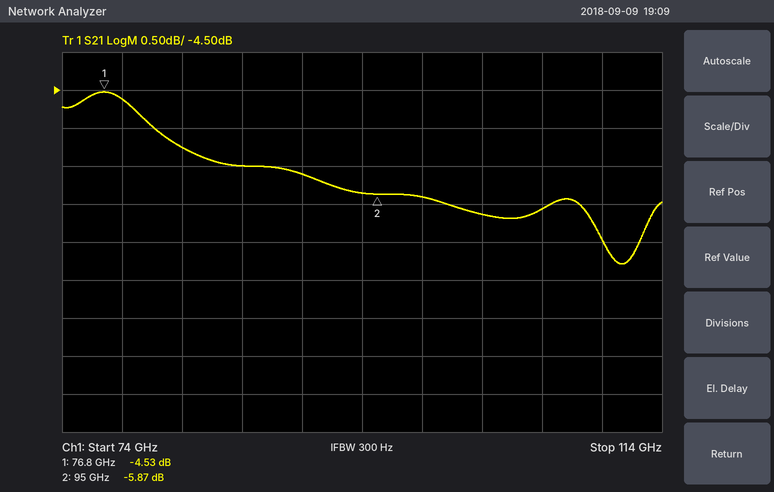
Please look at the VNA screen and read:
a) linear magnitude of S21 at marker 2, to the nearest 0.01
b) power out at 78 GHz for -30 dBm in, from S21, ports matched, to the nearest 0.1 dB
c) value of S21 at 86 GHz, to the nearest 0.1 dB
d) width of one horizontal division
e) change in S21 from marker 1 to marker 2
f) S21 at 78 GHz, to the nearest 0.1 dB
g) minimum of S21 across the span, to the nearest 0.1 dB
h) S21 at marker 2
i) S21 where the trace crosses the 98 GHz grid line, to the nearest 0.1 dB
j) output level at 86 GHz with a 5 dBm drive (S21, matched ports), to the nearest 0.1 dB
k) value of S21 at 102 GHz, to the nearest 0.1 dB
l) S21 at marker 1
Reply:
0.51
-34.6 dBm
-5.5 dB
4 GHz
-1.34 dB
-4.6 dB
-6.8 dB
-5.87 dB
-5.9 dB
-0.5 dBm
-6.1 dB
-4.53 dB
